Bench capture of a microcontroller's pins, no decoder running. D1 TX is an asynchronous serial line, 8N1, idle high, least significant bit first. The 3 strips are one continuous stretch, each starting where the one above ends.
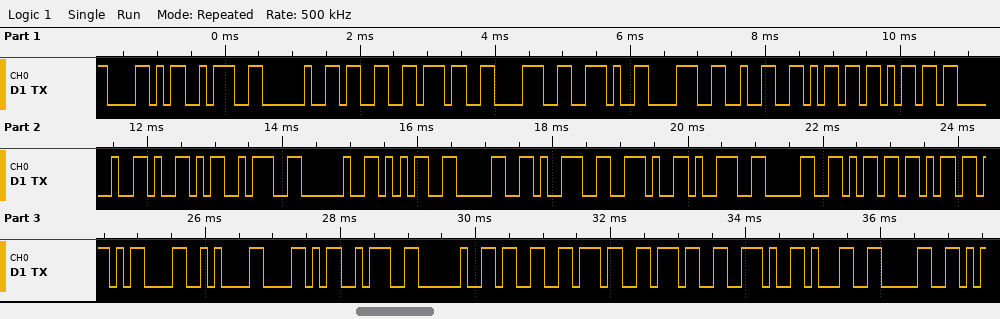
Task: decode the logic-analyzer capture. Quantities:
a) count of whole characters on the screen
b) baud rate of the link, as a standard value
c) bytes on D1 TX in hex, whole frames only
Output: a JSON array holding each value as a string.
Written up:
["34", "9600 baud", "0x58 0x3A 0x20 0x33 0x37 0x38 0x2E 0x38 0x32 0x6D 0x6D 0x20 0x59 0x3A 0x20 0x35 0x30 0x39 0x2E 0x39 0x30 0x6D 0x6D 0x0D 0x0A 0x58 0x3A 0x20 0x33 0x37 0x37 0x2E 0x31 0x30"]
